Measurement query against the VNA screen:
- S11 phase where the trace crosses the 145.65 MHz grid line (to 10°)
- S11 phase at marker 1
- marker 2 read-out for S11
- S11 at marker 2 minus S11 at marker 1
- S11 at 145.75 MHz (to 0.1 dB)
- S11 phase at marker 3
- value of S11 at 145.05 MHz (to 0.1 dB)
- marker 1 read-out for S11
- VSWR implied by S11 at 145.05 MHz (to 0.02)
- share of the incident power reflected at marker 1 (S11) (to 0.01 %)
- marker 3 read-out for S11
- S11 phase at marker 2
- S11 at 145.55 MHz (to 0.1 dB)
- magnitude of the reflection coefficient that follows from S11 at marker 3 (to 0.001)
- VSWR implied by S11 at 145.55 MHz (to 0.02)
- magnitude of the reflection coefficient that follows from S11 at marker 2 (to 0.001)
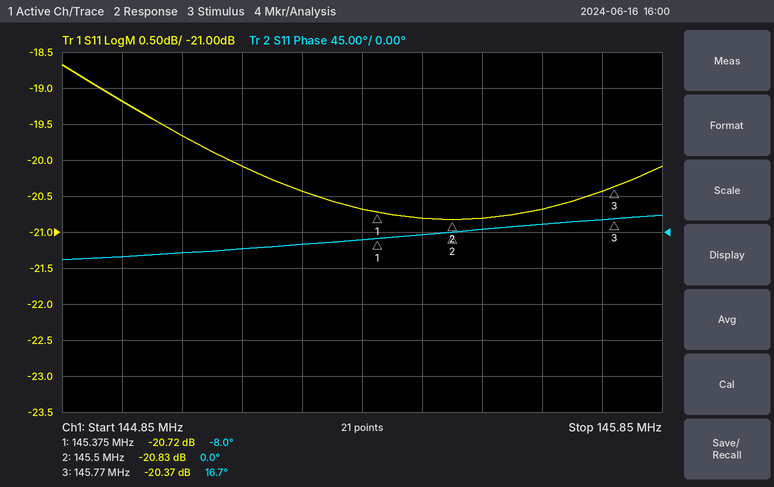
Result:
10°
-8.0°
-20.83 dB
-0.11 dB
-20.4 dB
16.7°
-19.7 dB
-20.72 dB
1.24
0.85 %
-20.37 dB
0.0°
-20.8 dB
0.096
1.20
0.091
